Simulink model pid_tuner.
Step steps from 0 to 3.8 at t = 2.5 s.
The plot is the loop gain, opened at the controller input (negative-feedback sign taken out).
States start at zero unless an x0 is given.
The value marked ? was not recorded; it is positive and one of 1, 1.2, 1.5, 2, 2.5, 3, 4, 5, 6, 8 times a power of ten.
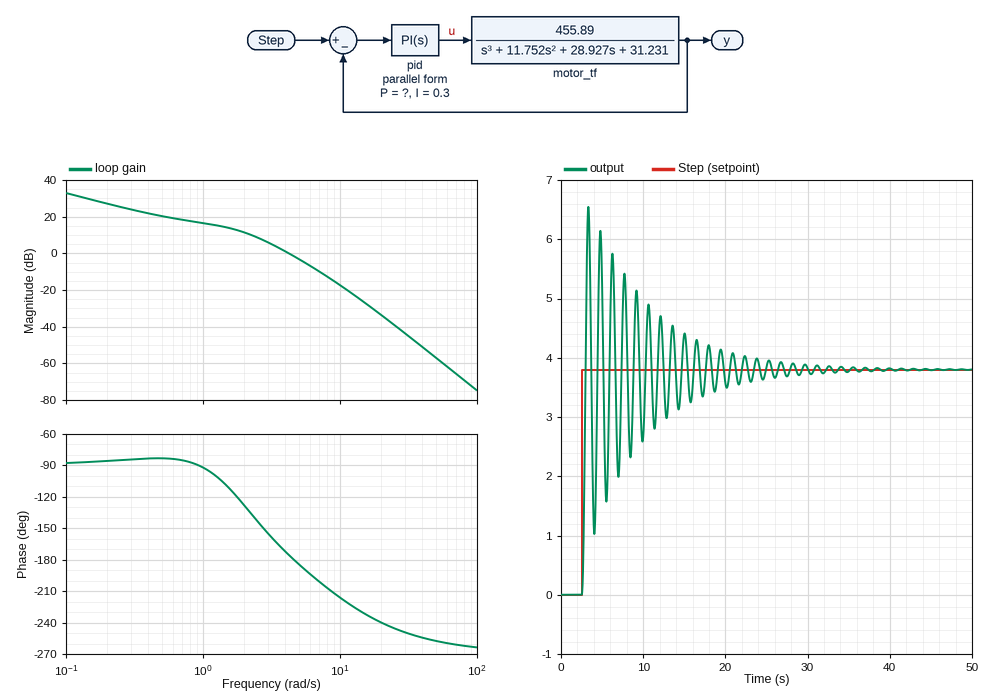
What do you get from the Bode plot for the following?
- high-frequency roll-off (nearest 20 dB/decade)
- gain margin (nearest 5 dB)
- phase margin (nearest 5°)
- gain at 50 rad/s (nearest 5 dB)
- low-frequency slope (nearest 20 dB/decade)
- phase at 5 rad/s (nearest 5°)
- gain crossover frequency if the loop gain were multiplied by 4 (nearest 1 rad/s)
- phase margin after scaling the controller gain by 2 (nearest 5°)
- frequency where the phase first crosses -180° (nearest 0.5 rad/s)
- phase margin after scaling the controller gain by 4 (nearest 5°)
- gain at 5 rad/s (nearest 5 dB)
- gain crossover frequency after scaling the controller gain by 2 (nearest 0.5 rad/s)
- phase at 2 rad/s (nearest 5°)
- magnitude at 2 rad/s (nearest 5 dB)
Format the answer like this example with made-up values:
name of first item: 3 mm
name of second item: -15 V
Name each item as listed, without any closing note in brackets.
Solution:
high-frequency roll-off: -60 dB/decade
gain margin: 0 dB
phase margin: 5°
gain at 50 rad/s: -55 dB
low-frequency slope: -20 dB/decade
phase at 5 rad/s: -185°
gain crossover frequency if the loop gain were multiplied by 4: 8 rad/s
phase margin after scaling the controller gain by 2: -10°
frequency where the phase first crosses -180°: 4.5 rad/s
phase margin after scaling the controller gain by 4: -25°
gain at 5 rad/s: -5 dB
gain crossover frequency after scaling the controller gain by 2: 6.0 rad/s
phase at 2 rad/s: -130°
magnitude at 2 rad/s: 10 dB
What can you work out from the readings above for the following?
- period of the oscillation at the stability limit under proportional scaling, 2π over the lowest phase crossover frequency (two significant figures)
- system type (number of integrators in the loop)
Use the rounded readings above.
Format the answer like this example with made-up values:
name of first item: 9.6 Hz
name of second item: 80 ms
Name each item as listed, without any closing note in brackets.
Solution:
period of the oscillation at the stability limit under proportional scaling, 2π over the lowest phase crossover frequency: 1.4 s
system type: 1
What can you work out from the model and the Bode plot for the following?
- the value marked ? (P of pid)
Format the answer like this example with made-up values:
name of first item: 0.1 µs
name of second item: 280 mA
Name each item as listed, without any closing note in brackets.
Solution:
the value marked ?: 0.4
